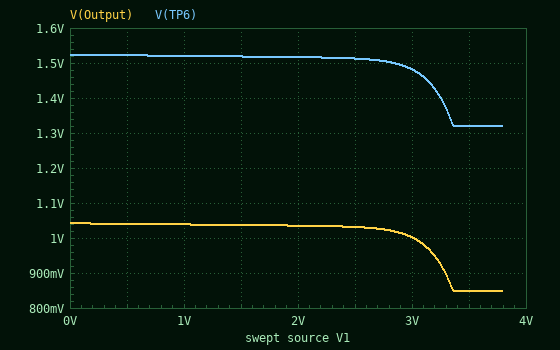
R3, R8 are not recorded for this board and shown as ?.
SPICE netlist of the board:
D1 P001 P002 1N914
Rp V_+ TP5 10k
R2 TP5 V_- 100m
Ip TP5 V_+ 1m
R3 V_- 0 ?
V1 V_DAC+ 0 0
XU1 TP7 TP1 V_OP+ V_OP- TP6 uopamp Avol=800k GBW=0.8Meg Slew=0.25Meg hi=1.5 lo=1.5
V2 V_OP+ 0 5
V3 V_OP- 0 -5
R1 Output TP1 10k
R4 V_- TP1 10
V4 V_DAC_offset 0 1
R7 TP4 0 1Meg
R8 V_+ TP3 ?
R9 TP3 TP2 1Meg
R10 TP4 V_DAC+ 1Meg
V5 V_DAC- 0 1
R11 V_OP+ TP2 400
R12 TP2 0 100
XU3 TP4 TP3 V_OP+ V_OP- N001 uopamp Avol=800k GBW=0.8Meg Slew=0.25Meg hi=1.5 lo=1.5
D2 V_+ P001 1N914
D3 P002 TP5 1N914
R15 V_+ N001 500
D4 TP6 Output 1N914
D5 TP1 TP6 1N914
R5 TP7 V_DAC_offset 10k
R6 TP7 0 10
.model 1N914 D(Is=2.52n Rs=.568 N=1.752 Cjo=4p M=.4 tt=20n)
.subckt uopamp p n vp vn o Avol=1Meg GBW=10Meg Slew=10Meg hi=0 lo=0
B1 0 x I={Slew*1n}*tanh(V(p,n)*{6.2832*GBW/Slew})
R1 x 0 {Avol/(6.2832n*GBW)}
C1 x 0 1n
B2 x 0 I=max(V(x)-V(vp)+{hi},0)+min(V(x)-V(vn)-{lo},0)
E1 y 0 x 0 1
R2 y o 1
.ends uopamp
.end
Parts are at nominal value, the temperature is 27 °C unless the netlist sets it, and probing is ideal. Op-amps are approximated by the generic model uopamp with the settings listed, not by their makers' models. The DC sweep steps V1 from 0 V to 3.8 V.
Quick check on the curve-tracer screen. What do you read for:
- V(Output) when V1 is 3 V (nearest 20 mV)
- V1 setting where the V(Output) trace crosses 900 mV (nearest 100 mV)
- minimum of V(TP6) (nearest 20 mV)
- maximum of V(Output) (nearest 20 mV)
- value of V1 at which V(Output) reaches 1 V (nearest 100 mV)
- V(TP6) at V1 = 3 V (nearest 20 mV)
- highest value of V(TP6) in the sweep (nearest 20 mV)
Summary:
1.00 V
3.3 V
1.32 V
1.04 V
3.0 V
1.48 V
1.52 V
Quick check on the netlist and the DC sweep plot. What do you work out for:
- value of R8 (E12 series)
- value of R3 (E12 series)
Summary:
390 kΩ
0.047 Ω
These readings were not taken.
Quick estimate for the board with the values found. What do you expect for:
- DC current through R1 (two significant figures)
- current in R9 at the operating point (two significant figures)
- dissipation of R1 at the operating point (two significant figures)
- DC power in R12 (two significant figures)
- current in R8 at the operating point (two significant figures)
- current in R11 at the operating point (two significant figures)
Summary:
100 µA
1.0 µA
110 µW
10 mW
1.0 µA
10 mA
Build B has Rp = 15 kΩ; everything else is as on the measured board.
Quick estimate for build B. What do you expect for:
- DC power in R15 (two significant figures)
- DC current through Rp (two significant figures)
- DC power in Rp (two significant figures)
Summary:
530 µW
26 µA
10 µW
